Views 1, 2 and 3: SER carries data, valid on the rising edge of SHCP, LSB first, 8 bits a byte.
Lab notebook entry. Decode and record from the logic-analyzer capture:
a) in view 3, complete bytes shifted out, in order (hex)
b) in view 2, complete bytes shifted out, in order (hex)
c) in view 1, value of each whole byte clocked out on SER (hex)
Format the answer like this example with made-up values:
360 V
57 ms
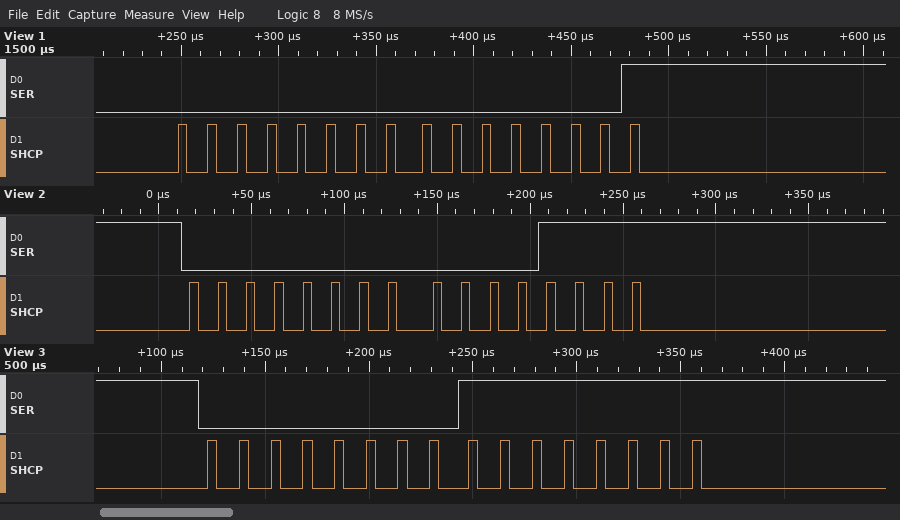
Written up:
00 FF
00 F0
00 80
